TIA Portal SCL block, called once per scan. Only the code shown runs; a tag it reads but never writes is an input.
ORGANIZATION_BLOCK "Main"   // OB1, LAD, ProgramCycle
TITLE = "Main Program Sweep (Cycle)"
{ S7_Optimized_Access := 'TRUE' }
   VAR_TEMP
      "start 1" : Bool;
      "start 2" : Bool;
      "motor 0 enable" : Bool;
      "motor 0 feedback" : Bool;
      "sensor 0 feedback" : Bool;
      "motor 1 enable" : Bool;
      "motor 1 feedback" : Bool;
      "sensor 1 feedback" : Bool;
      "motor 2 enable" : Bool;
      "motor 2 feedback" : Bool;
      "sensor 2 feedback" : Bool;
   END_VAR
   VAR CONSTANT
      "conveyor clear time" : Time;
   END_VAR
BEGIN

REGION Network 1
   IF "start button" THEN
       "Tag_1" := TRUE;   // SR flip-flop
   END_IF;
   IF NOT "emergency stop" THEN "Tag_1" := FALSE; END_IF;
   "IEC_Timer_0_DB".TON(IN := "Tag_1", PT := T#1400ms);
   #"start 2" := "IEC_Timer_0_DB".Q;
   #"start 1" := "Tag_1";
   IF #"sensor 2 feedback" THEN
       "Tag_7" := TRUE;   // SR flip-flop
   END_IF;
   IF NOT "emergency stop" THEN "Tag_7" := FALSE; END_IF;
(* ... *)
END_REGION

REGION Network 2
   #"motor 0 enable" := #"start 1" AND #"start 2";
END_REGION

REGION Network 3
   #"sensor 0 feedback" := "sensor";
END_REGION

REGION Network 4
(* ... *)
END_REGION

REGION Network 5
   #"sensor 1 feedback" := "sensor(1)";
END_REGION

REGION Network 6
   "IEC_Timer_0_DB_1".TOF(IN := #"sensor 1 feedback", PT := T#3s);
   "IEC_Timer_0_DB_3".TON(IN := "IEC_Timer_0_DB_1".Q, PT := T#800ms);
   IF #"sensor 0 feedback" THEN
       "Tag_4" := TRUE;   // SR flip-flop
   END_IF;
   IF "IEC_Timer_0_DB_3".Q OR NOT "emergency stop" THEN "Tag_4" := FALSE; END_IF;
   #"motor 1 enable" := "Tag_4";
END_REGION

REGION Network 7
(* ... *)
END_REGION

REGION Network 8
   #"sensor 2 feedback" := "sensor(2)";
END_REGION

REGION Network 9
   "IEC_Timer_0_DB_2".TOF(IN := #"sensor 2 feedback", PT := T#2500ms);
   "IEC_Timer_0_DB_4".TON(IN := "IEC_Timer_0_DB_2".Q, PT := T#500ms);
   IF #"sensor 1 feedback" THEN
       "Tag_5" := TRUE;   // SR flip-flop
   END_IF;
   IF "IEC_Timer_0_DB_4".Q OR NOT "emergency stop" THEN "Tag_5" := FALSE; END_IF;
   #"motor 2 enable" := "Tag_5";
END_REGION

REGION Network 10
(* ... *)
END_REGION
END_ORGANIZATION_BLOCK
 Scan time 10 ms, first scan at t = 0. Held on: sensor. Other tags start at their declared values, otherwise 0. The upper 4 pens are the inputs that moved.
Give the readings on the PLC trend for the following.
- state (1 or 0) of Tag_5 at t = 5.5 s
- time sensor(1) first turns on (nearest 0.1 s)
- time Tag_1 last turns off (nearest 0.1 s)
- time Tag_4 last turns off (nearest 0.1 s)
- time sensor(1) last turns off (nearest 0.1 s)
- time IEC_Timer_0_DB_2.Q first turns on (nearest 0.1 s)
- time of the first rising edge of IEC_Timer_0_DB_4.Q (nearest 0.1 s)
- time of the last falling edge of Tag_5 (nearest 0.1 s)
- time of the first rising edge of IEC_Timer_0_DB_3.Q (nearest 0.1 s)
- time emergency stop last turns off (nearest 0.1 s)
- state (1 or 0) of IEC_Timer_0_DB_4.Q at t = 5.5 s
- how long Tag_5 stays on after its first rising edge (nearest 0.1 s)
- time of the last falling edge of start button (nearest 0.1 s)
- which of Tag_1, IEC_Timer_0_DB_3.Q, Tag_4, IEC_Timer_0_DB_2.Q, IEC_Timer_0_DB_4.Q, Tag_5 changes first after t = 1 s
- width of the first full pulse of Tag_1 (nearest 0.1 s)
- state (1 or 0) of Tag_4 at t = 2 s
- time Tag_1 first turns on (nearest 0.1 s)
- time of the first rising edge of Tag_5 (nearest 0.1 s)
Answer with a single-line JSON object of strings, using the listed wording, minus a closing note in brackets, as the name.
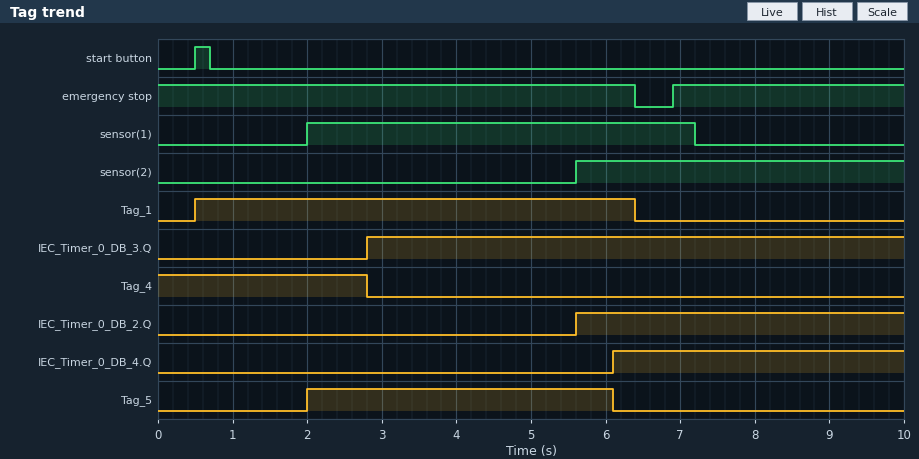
{"state (1 or 0) of Tag_5 at t = 5.5 s": "1", "time sensor(1) first turns on": "2.0 s", "time Tag_1 last turns off": "6.4 s", "time Tag_4 last turns off": "2.8 s", "time sensor(1) last turns off": "7.2 s", "time IEC_Timer_0_DB_2.Q first turns on": "5.6 s", "time of the first rising edge of IEC_Timer_0_DB_4.Q": "6.1 s", "time of the last falling edge of Tag_5": "6.1 s", "time of the first rising edge of IEC_Timer_0_DB_3.Q": "2.8 s", "time emergency stop last turns off": "6.4 s", "state (1 or 0) of IEC_Timer_0_DB_4.Q at t = 5.5 s": "0", "how long Tag_5 stays on after its first rising edge": "4.1 s", "time of the last falling edge of start button": "0.7 s", "which of Tag_1, IEC_Timer_0_DB_3.Q, Tag_4, IEC_Timer_0_DB_2.Q, IEC_Timer_0_DB_4.Q, Tag_5 changes first after t = 1 s": "Tag_5", "width of the first full pulse of Tag_1": "5.9 s", "state (1 or 0) of Tag_4 at t = 2 s": "1", "time Tag_1 first turns on": "0.5 s", "time of the first rising edge of Tag_5": "2.0 s"}
